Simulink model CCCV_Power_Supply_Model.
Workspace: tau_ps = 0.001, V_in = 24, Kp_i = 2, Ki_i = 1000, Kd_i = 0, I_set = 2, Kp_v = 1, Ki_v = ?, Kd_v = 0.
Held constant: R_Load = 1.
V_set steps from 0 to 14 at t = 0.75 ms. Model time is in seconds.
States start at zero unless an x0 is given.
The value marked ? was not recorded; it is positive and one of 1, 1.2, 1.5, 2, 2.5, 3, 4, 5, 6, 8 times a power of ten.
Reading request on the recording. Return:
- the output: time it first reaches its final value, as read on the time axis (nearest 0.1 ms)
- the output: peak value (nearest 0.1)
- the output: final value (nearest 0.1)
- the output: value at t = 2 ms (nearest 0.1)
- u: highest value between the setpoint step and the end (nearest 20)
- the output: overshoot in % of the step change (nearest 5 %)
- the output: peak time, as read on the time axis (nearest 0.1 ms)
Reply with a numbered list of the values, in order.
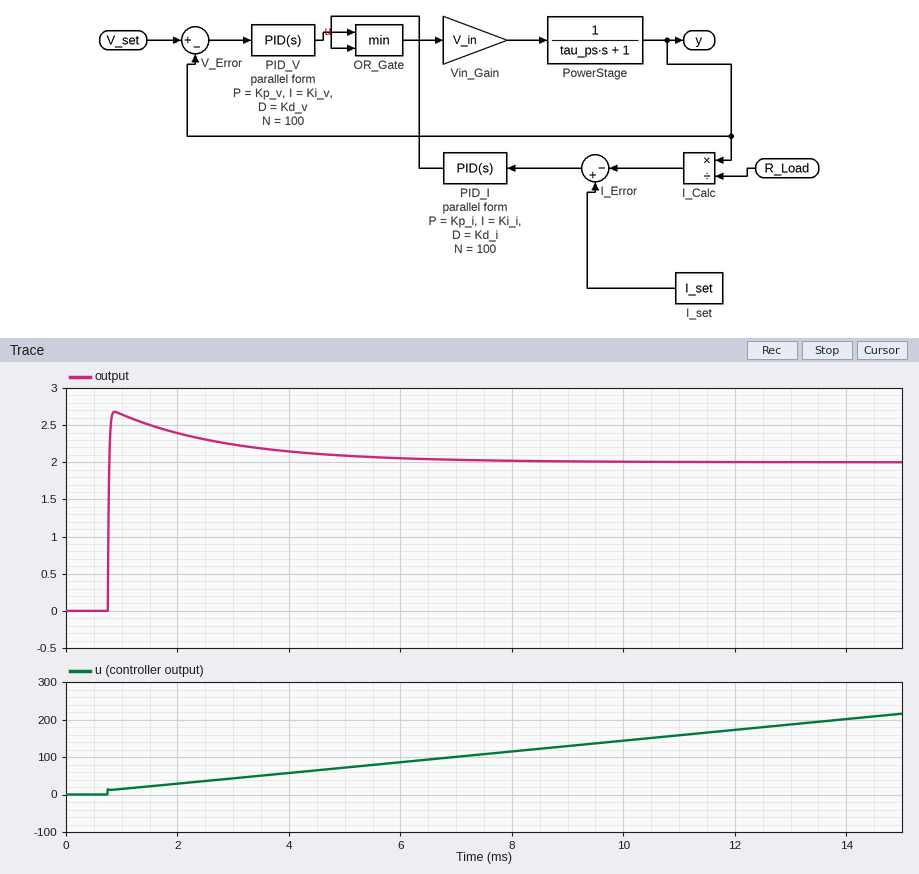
1. 0.8 ms
2. 2.7
3. 2.0
4. 2.4
5. 220
6. 35 %
7. 0.9 ms
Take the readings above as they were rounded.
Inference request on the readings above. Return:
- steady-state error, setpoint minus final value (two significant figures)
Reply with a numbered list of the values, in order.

1. 12
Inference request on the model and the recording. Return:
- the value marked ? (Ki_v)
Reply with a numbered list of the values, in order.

1. 1200
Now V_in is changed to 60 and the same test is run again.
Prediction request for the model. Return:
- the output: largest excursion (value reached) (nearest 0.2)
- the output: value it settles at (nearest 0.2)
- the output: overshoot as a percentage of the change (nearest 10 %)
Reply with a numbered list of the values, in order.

1. 2.8
2. 2.0
3. 40 %
